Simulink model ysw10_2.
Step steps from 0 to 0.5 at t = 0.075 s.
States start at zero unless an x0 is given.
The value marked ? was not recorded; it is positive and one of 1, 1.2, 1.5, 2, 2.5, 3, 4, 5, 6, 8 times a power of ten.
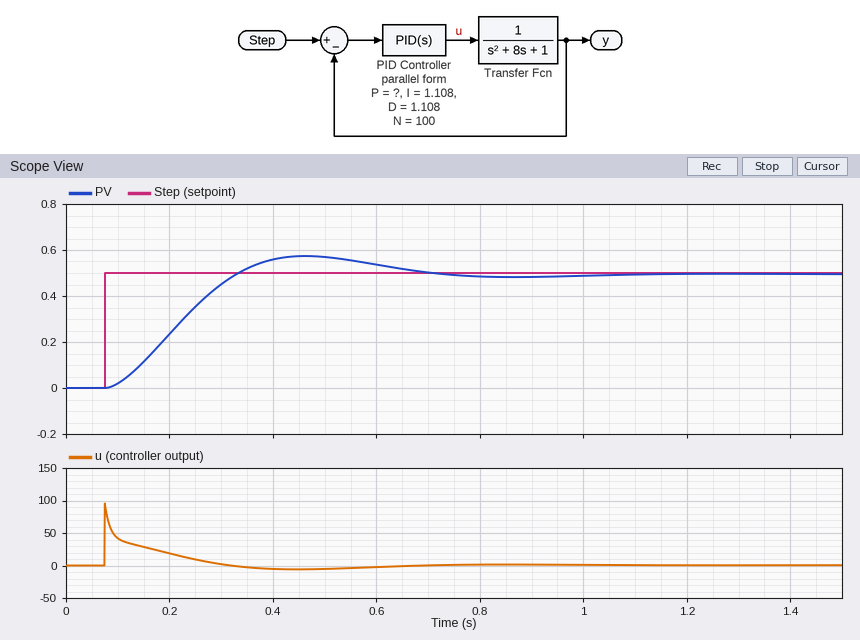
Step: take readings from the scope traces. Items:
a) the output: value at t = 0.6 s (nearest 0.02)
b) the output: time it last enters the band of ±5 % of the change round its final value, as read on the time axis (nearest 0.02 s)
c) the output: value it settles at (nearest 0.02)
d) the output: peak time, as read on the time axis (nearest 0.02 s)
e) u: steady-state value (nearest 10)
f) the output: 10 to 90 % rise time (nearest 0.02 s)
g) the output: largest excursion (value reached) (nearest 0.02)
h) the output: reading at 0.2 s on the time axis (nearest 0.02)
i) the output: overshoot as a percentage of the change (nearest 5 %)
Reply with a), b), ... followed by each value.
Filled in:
a) 0.54
b) 0.64 s
c) 0.50
d) 0.46 s
e) 0
f) 0.18 s
g) 0.58
h) 0.24
i) 15 %
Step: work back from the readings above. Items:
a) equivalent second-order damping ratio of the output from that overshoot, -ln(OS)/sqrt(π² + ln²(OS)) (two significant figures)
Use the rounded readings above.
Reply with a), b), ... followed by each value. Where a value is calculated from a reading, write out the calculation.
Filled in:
a) ln(0.15) = -1.897; 1.897 / sqrt(9.870 + 3.599) = 0.52
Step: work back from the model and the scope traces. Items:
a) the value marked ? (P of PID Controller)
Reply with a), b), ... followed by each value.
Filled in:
a) 80
